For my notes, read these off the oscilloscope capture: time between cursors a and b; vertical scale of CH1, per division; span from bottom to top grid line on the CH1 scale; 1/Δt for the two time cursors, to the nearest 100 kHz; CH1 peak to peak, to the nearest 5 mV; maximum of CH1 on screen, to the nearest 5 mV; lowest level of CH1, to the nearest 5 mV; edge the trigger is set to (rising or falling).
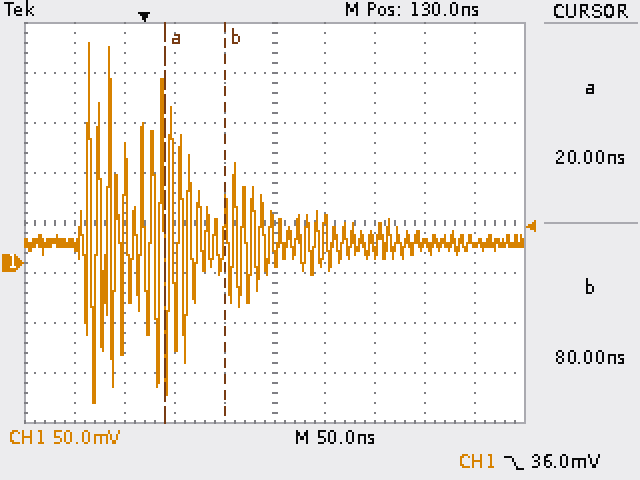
60 ns
50 mV
400 mV
16.7 MHz
360 mV
220 mV
-140 mV
falling
